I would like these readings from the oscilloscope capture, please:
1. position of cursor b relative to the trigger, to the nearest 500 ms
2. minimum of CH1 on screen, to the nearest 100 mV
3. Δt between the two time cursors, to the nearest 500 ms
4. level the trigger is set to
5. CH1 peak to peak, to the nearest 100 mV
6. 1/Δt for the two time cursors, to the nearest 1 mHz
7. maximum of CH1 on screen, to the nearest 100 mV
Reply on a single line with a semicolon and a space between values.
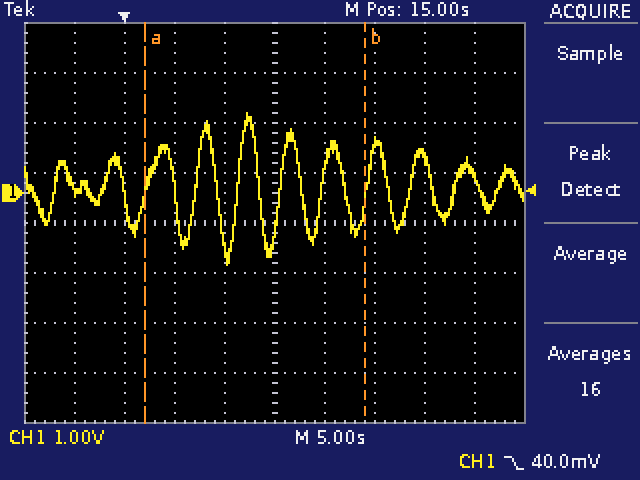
+24.0 s; -1.4 V; 22.0 s; 40.0 mV; 3.0 V; 45 mHz; 1.6 V
